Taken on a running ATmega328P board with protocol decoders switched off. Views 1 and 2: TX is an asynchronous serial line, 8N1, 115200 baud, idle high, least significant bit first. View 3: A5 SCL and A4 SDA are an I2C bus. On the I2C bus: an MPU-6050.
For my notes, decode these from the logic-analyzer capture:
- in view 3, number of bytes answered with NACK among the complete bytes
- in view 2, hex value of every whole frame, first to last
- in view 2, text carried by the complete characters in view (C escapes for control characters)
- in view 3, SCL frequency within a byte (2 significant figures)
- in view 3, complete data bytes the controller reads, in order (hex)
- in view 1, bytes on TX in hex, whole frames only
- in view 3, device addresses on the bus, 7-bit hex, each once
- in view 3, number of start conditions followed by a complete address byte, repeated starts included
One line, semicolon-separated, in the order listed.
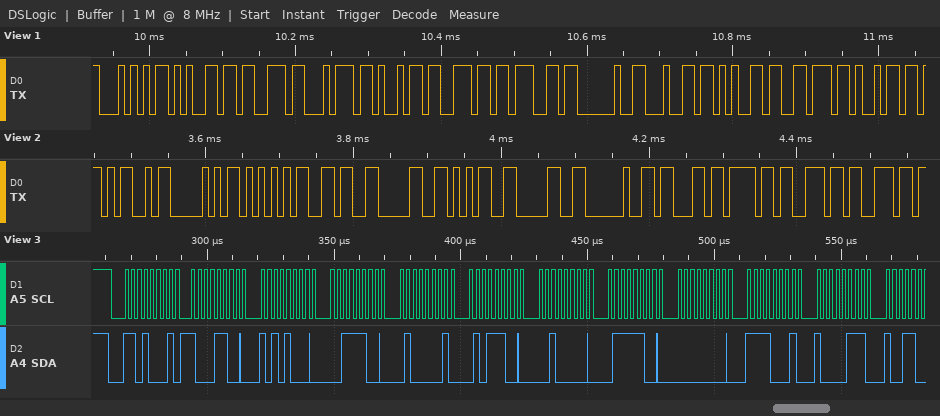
0; 4D 50 55 36 30 35 30 20 63 6F 6E 6E; "MPU6050 conn"; 400 kHz; 8C A8 3C 41 5C 20 7C 00 F1 87; 0x54 0x65 0x73 0x74 0x69 0x6E 0x67 0x20 0x64 0x65 0x76 0x69; 0x68; 1
